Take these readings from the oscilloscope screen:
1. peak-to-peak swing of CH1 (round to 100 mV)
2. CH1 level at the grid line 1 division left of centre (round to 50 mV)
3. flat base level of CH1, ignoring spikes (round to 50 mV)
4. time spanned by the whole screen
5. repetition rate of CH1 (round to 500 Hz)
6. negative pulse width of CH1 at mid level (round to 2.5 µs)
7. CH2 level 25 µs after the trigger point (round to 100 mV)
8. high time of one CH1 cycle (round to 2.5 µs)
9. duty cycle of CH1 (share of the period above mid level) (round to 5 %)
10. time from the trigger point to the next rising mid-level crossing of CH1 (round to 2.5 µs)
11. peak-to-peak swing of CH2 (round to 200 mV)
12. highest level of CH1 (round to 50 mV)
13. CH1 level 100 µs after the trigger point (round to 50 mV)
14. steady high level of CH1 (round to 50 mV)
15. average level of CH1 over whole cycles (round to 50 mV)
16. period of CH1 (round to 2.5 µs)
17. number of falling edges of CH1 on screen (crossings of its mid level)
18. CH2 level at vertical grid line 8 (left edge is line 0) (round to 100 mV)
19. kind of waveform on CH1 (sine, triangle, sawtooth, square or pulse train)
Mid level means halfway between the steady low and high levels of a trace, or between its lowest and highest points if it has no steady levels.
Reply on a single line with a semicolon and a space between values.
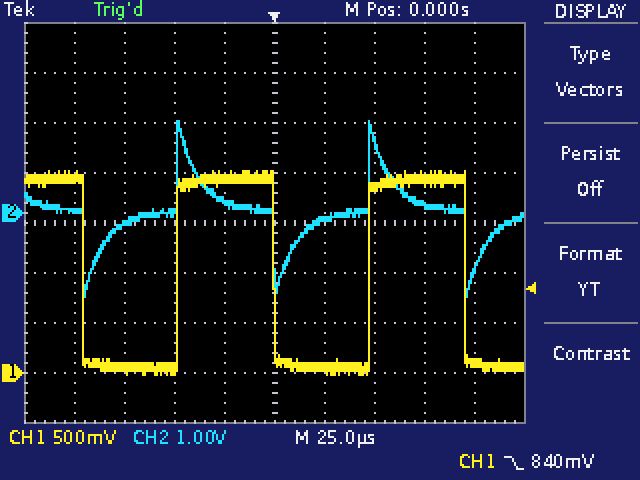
2.00 V; 1.95 V; 50 mV; 250 µs; 10.5 kHz; 47.5 µs; -100 mV; 47.5 µs; 50 %; 47.5 µs; 3.6 V; 2.00 V; 100 mV; 1.95 V; 1.00 V; 95.0 µs; 3; 200 mV; square
